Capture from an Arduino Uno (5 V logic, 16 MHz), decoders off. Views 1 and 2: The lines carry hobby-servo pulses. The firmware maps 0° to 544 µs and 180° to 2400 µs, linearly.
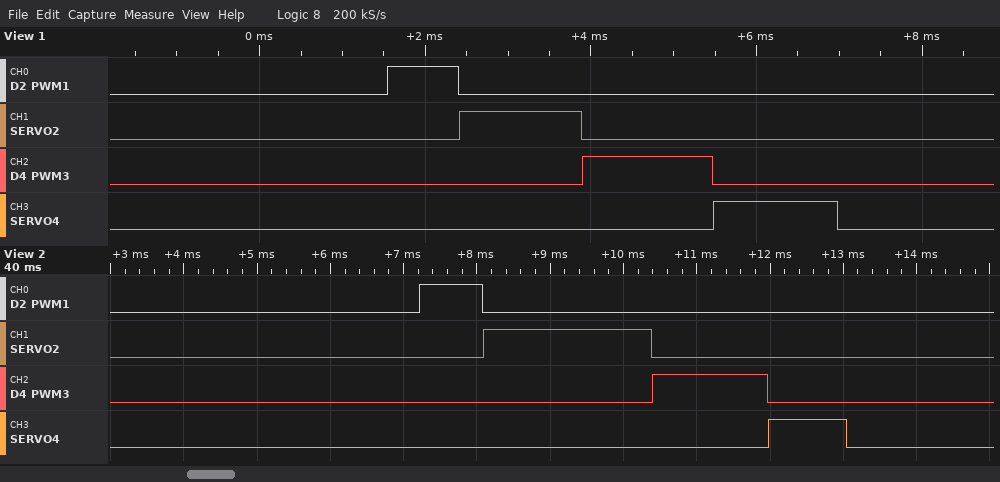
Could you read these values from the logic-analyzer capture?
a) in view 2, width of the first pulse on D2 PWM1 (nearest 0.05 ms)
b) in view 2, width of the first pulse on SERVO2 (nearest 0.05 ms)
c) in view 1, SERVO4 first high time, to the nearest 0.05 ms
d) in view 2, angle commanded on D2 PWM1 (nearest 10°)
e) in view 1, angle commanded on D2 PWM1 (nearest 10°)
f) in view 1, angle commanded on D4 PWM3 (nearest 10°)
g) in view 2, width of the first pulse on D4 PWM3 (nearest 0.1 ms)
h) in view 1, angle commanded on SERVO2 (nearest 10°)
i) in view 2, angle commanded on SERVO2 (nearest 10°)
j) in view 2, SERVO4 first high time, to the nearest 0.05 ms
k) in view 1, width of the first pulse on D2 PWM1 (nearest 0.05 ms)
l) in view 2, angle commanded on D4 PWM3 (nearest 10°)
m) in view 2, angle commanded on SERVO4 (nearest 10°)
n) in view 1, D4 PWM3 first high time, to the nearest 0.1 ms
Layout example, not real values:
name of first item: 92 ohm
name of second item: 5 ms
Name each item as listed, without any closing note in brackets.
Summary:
in view 2, width of the first pulse on D2 PWM1: 0.85 ms
in view 2, width of the first pulse on SERVO2: 2.30 ms
in view 1, SERVO4 first high time, to the nearest 0.05 ms: 1.50 ms
in view 2, angle commanded on D2 PWM1: 30°
in view 1, angle commanded on D2 PWM1: 30°
in view 1, angle commanded on D4 PWM3: 100°
in view 2, width of the first pulse on D4 PWM3: 1.6 ms
in view 1, angle commanded on SERVO2: 90°
in view 2, angle commanded on SERVO2: 170°
in view 2, SERVO4 first high time, to the nearest 0.05 ms: 1.05 ms
in view 1, width of the first pulse on D2 PWM1: 0.85 ms
in view 2, angle commanded on D4 PWM3: 100°
in view 2, angle commanded on SERVO4: 50°
in view 1, D4 PWM3 first high time, to the nearest 0.1 ms: 1.6 ms
